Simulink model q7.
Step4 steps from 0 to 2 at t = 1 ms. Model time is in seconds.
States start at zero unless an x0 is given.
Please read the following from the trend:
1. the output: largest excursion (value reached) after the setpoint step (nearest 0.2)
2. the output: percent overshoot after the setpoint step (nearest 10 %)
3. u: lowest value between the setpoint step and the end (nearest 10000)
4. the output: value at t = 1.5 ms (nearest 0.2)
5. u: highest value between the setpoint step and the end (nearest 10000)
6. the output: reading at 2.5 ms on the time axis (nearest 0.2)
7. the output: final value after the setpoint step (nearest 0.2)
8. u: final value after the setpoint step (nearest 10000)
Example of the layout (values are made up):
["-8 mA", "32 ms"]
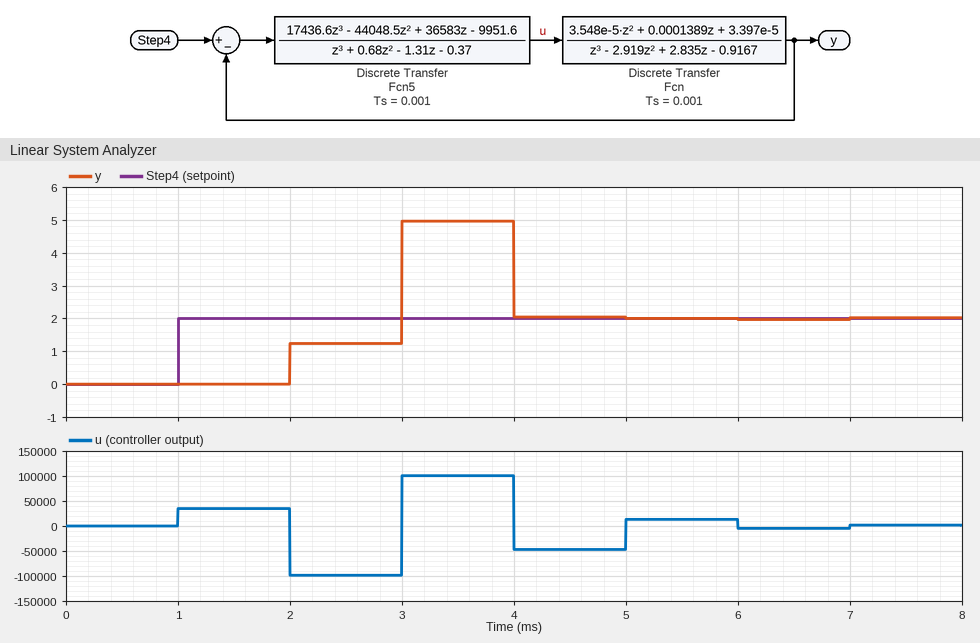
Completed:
["5.0", "150 %", "-100000", "0.0", "100000", "1.2", "2.0", "0"]
